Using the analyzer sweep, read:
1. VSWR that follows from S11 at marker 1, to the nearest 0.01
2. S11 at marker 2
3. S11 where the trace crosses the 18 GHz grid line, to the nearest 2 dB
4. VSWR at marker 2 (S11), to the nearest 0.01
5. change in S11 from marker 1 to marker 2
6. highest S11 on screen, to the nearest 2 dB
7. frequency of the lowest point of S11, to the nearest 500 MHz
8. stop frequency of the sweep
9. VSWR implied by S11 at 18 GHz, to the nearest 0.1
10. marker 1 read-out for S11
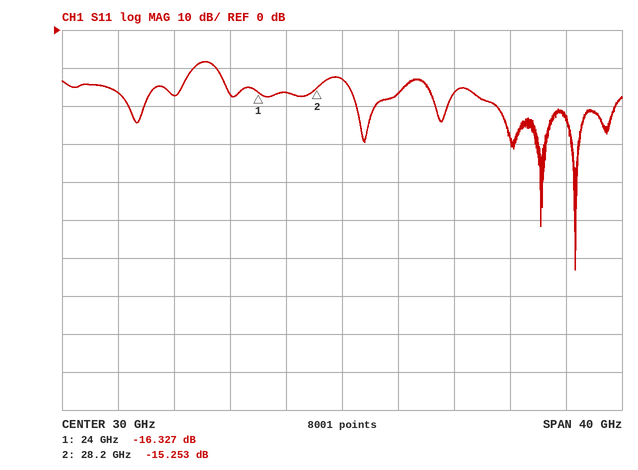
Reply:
1.36
-15.253 dB
-18 dB
1.42
1.074 dB
-8 dB
46.5 GHz
50 GHz
1.3
-16.327 dB
